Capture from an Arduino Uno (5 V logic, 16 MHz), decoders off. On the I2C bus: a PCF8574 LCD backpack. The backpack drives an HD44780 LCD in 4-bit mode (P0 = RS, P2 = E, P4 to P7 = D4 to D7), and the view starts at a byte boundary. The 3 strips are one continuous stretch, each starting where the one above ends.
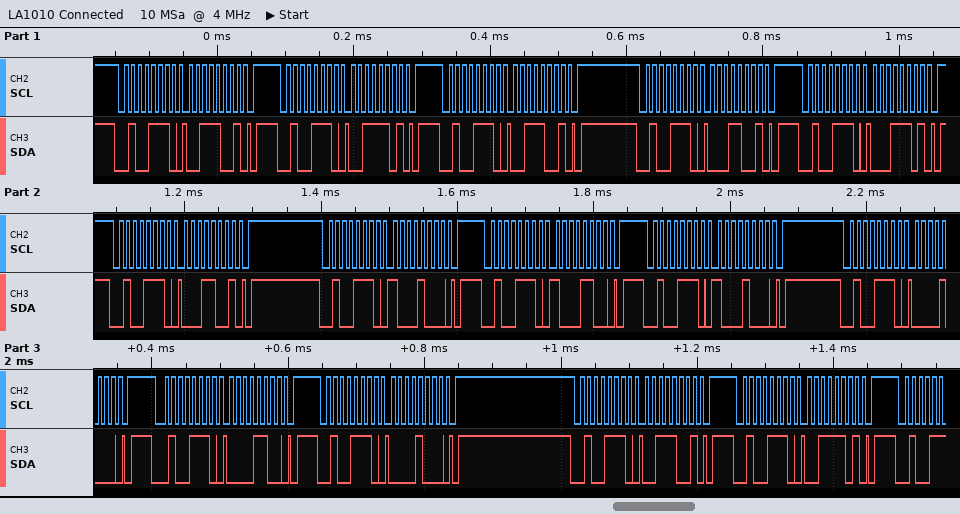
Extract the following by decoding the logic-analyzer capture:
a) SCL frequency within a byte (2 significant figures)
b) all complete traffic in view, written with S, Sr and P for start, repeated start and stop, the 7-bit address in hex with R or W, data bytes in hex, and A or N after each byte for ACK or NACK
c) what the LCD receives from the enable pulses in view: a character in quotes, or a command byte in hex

100 kHz
S 27W A 39 A P S 27W A 3D A P S 27W A 39 A P S 27W A 19 A P S 27W A 1D A P S 27W A 19 A P S 27W A 88 A P S 27W A 8C A P S 27W A 88 A P S 27W A 08 A P S 27W A 0C A P S 27W A 08 A P S 27W A 39 A P S 27W A 3D A P
'1' 0x80
